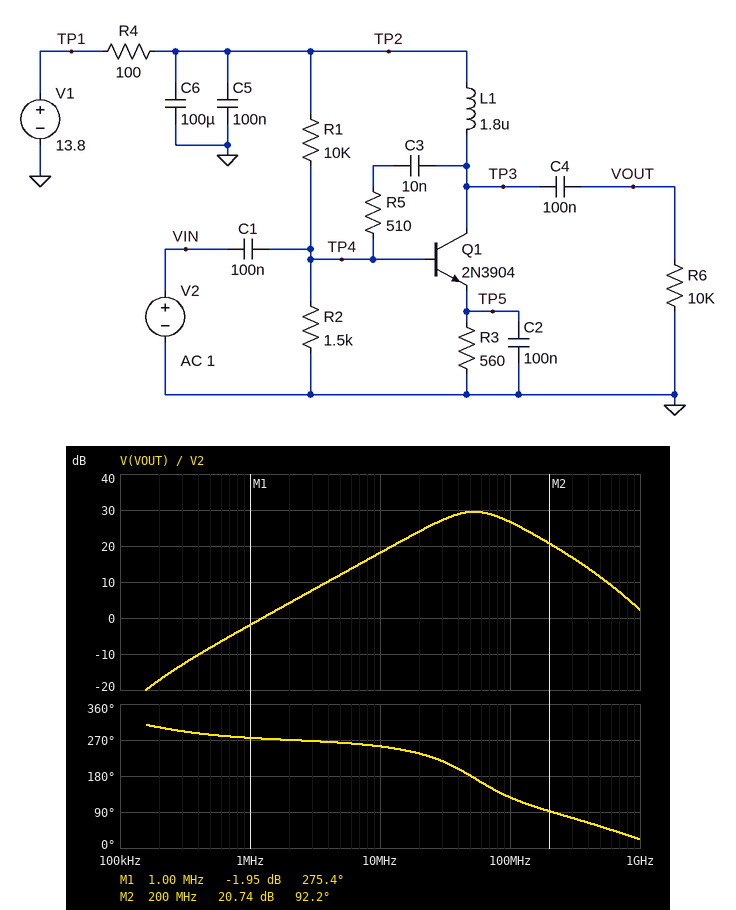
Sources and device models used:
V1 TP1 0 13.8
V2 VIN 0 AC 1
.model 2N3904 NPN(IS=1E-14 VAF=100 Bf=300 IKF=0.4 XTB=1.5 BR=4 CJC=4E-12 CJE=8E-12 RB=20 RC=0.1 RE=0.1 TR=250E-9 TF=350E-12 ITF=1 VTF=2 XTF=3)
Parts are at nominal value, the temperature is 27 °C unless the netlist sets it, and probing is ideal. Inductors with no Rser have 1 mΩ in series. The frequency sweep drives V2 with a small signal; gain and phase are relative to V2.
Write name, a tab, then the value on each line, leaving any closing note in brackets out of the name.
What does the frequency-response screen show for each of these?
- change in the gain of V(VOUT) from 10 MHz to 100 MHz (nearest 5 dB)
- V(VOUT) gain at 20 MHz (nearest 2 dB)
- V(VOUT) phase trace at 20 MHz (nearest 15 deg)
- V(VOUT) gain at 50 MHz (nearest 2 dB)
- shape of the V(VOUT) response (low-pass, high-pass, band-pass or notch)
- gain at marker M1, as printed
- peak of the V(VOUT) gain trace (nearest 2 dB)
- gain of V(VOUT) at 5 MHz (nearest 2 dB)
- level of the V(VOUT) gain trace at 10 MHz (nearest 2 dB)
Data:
change in the gain of V(VOUT) from 10 MHz to 100 MHz	10 dB
V(VOUT) gain at 20 MHz	24 dB
V(VOUT) phase trace at 20 MHz	240 deg
V(VOUT) gain at 50 MHz	30 dB
shape of the V(VOUT) response	band-pass
gain at marker M1, as printed	-1.95 dB
peak of the V(VOUT) gain trace	30 dB
gain of V(VOUT) at 5 MHz	12 dB
level of the V(VOUT) gain trace at 10 MHz	18 dB
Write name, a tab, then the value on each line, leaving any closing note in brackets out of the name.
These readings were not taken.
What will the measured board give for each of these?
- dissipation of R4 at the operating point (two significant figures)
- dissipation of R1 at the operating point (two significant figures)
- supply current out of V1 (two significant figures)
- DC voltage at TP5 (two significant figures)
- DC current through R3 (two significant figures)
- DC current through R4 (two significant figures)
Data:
dissipation of R4 at the operating point	960 µW
dissipation of R1 at the operating point	14 mW
supply current out of V1	3.1 mA
DC voltage at TP5	1.1 V
DC current through R3	1.9 mA
DC current through R4	3.1 mA
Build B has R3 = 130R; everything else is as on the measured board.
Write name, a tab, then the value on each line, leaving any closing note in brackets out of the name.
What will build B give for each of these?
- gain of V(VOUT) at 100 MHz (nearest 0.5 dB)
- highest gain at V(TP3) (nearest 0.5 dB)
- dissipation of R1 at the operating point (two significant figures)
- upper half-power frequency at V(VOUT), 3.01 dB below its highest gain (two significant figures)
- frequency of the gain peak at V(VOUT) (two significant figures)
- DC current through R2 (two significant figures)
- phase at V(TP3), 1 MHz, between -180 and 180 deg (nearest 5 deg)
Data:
gain of V(VOUT) at 100 MHz	30.0 dB
highest gain at V(TP3)	38.5 dB
dissipation of R1 at the operating point	13 mW
upper half-power frequency at V(VOUT), 3.01 dB below its highest gain	55 MHz
frequency of the gain peak at V(VOUT)	32 MHz
DC current through R2	1.1 mA
phase at V(TP3), 1 MHz, between -180 and 180 deg	-70 deg
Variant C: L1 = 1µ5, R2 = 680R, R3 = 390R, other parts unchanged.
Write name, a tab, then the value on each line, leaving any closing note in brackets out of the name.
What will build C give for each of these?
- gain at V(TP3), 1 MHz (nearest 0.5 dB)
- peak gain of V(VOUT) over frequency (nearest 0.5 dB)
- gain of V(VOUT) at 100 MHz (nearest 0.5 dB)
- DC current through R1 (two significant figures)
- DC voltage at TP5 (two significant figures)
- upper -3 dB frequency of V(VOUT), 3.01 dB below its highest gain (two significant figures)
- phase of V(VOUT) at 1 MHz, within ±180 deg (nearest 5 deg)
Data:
gain at V(TP3), 1 MHz	-14.5 dB
peak gain of V(VOUT) over frequency	19.5 dB
gain of V(VOUT) at 100 MHz	19.0 dB
DC current through R1	1.3 mA
DC voltage at TP5	230 mV
upper -3 dB frequency of V(VOUT), 3.01 dB below its highest gain	170 MHz
phase of V(VOUT) at 1 MHz, within ±180 deg	-90 deg
